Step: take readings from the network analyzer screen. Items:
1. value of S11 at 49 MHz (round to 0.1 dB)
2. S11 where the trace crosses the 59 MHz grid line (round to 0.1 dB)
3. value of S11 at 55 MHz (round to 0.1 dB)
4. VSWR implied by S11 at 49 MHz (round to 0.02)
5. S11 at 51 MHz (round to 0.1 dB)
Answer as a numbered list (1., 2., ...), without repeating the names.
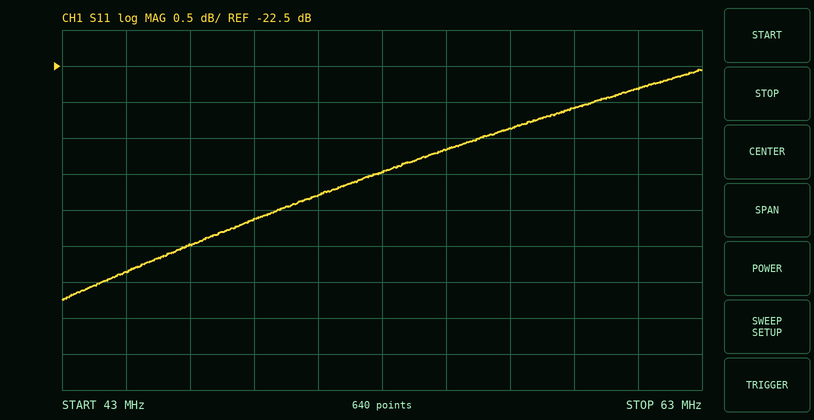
1. -24.6 dB
2. -23.1 dB
3. -23.7 dB
4. 1.12
5. -24.3 dB
